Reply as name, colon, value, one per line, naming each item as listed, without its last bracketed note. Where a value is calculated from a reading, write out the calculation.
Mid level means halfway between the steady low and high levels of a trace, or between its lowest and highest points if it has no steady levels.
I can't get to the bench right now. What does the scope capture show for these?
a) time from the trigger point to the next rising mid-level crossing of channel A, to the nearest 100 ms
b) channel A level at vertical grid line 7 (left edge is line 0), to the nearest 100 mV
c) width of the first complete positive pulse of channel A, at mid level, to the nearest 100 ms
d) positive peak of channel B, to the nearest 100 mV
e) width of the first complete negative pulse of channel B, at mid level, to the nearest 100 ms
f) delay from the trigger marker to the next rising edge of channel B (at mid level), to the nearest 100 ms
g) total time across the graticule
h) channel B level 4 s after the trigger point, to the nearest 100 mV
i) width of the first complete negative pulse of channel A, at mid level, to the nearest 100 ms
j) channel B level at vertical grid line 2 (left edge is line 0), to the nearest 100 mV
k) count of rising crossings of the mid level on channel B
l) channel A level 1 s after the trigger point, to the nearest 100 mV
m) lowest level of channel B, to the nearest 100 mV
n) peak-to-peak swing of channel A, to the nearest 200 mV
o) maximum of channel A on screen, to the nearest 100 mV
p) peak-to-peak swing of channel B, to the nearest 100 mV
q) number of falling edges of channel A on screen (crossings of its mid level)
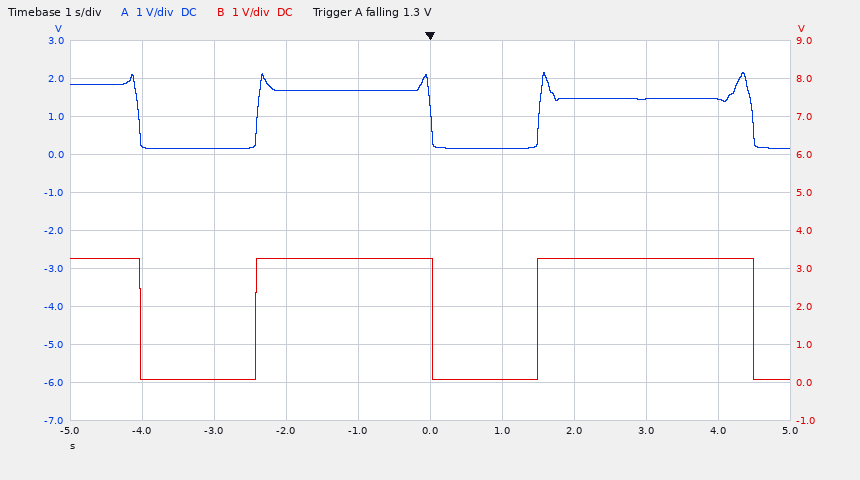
time from the trigger point to the next rising mid-level crossing of channel A, to the nearest 100 ms: 1.5 s
channel A level at vertical grid line 7 (left edge is line 0), to the nearest 100 mV: 1.5 V
width of the first complete positive pulse of channel A, at mid level, to the nearest 100 ms: 2.4 s
positive peak of channel B, to the nearest 100 mV: 3.3 V
width of the first complete negative pulse of channel B, at mid level, to the nearest 100 ms: 1.6 s
delay from the trigger marker to the next rising edge of channel B (at mid level), to the nearest 100 ms: 1.5 s
total time across the graticule: 10 s
channel B level 4 s after the trigger point, to the nearest 100 mV: 3.3 V
width of the first complete negative pulse of channel A, at mid level, to the nearest 100 ms: 1.7 s
channel B level at vertical grid line 2 (left edge is line 0), to the nearest 100 mV: 100 mV
count of rising crossings of the mid level on channel B: 2
channel A level 1 s after the trigger point, to the nearest 100 mV: 200 mV
lowest level of channel B, to the nearest 100 mV: 100 mV
peak-to-peak swing of channel A, to the nearest 200 mV: 2.0 V
maximum of channel A on screen, to the nearest 100 mV: 2.2 V
peak-to-peak swing of channel B, to the nearest 100 mV: 3.3 V − (100 mV) = 3.2 V
number of falling edges of channel A on screen: 3
